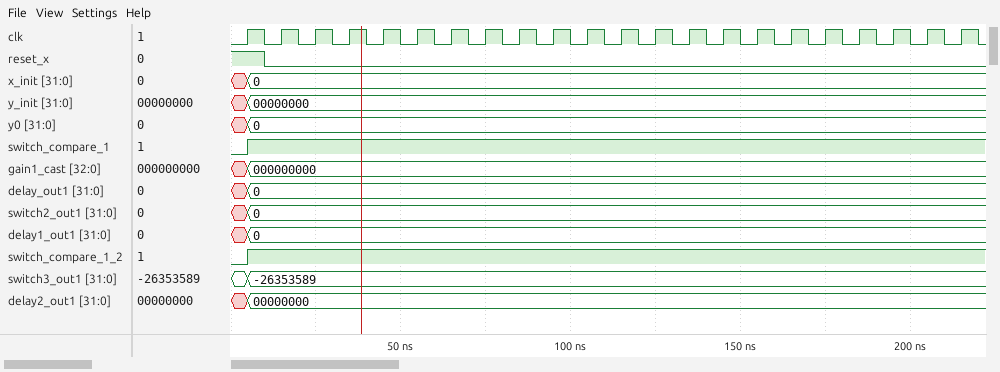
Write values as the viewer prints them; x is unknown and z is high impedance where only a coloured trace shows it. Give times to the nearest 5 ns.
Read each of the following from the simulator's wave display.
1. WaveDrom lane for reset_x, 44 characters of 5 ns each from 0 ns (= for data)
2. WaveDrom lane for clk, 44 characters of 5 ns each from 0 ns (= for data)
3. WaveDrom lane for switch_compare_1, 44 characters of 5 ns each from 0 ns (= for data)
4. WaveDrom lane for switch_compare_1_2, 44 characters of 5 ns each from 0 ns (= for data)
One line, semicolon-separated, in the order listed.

{name: 'reset_x', wave: '1.0.........................................'}; {name: 'clk', wave: '01010101010101010101010101010101010101010101'}; {name: 'switch_compare_1', wave: '01..........................................'}; {name: 'switch_compare_1_2', wave: '01..........................................'}
